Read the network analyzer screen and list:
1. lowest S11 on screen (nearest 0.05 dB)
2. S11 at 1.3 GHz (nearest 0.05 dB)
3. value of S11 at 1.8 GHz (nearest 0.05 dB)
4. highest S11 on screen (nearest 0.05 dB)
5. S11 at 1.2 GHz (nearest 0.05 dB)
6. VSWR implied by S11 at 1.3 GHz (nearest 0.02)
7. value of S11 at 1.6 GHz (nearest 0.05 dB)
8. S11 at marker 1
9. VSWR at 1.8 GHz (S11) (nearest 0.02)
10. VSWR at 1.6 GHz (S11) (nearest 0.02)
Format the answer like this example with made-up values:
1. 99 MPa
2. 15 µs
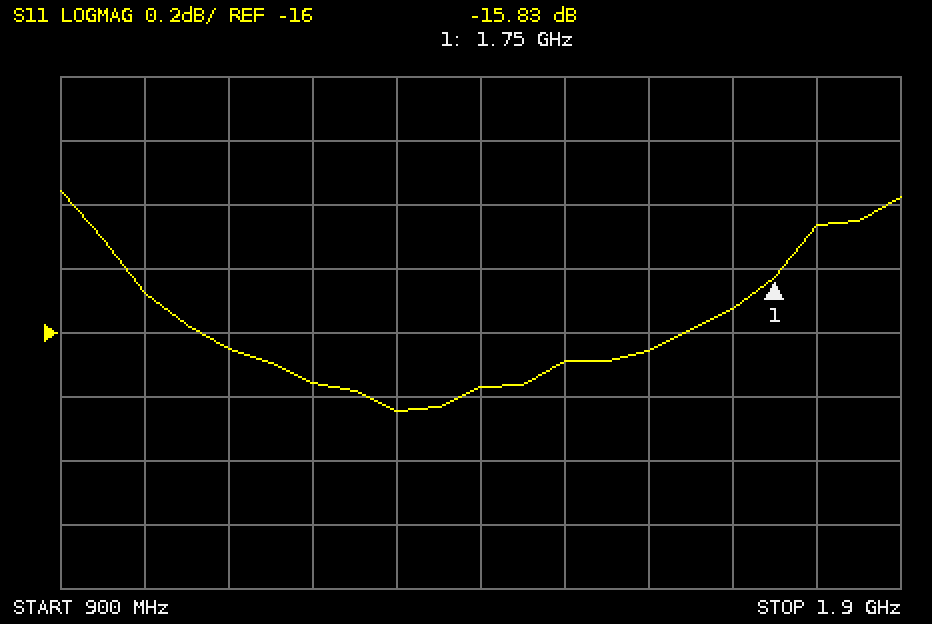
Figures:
1. -16.25 dB
2. -16.25 dB
3. -15.65 dB
4. -15.55 dB
5. -16.15 dB
6. 1.36
7. -16.05 dB
8. -15.83 dB
9. 1.40
10. 1.38
